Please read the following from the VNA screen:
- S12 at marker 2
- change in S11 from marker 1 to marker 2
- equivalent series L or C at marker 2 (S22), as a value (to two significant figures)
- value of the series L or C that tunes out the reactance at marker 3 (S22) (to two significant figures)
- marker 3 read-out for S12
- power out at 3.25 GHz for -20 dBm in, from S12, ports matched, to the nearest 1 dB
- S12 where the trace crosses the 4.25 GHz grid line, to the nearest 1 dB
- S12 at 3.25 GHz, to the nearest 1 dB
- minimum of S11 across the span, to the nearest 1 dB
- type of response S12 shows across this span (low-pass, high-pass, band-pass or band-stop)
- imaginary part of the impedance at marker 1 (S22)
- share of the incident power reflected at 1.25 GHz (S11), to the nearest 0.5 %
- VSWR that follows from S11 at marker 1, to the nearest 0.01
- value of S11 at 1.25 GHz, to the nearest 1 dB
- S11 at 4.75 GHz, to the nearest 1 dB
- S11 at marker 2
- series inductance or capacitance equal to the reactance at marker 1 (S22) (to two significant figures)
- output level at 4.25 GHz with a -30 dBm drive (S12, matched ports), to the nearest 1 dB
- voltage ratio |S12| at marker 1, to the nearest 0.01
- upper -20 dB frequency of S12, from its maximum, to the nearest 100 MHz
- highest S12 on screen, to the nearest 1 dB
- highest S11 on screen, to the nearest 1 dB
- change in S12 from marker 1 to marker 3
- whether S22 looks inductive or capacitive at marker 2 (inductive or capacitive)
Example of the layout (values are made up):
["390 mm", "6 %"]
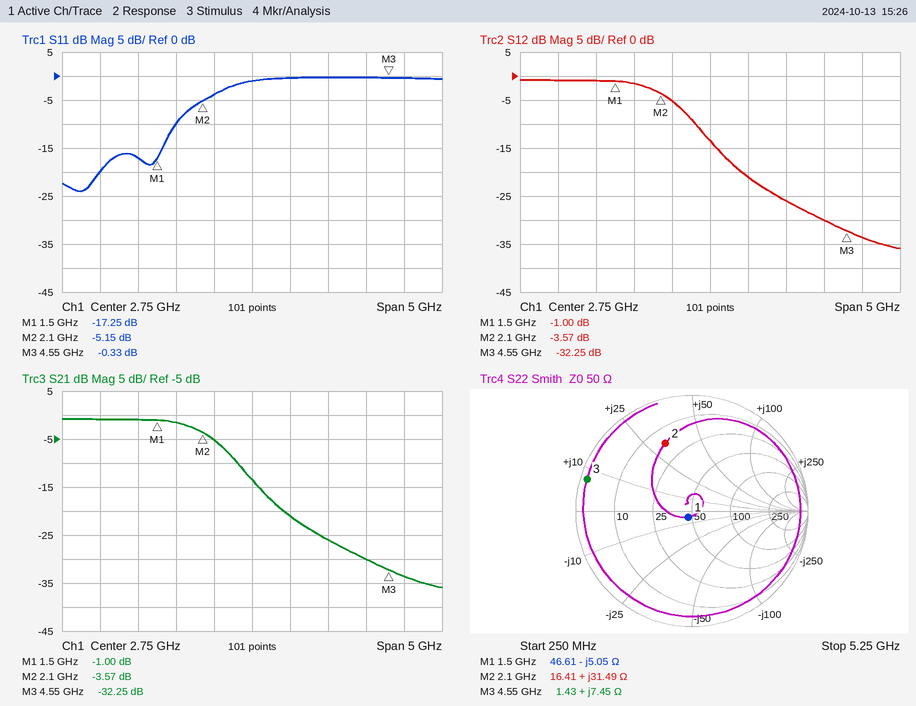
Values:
["-3.57 dB", "12.10 dB", "2.4 nH", "4.7 pF", "-32.25 dB", "-41 dBm", "-30 dB", "-21 dB", "-24 dB", "low-pass", "-5.05 Ω", "2.0 %", "1.32", "-17 dB", "0 dB", "-5.15 dB", "21 pF", "-60 dBm", "0.89", "3.2 GHz", "-1 dB", "0 dB", "-31.25 dB", "inductive"]
